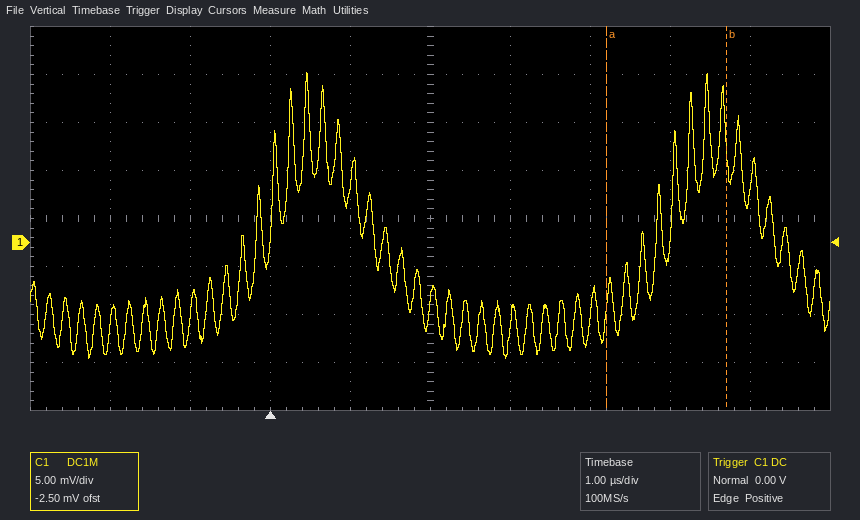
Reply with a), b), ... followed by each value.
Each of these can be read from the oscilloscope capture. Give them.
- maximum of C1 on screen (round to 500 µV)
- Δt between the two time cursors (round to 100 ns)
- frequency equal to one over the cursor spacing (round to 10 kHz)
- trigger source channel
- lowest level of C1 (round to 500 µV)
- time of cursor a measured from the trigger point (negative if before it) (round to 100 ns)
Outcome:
a) 17.5 mV
b) 1.5 µs
c) 670 kHz
d) C1
e) -12.0 mV
f) +4.2 µs
